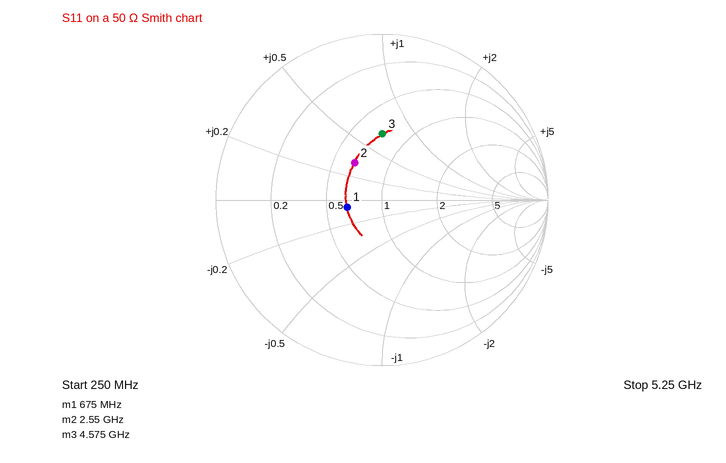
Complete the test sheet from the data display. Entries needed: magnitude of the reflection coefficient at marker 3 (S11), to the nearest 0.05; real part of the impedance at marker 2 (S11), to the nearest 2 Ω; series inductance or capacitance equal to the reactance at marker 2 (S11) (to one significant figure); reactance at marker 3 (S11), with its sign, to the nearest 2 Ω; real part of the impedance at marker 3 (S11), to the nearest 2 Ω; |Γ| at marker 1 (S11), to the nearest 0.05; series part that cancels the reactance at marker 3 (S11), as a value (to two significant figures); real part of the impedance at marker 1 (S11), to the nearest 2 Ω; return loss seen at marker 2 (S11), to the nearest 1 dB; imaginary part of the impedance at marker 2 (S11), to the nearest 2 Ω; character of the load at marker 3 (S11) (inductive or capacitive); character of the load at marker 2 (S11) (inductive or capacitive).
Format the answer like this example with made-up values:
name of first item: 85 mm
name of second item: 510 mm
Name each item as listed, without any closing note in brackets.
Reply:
magnitude of the reflection coefficient at marker 3 (S11), to the nearest 0.05: 0.40
real part of the impedance at marker 2 (S11), to the nearest 2 Ω: 32 Ω
series inductance or capacitance equal to the reactance at marker 2 (S11): 1.0 nH
reactance at marker 3 (S11), with its sign, to the nearest 2 Ω: +34 Ω
real part of the impedance at marker 3 (S11), to the nearest 2 Ω: 36 Ω
|Γ| at marker 1 (S11), to the nearest 0.05: 0.20
series part that cancels the reactance at marker 3 (S11), as a value: 1.0 pF
real part of the impedance at marker 1 (S11), to the nearest 2 Ω: 32 Ω
return loss seen at marker 2 (S11), to the nearest 1 dB: 11 dB
imaginary part of the impedance at marker 2 (S11), to the nearest 2 Ω: +16 Ω
character of the load at marker 3 (S11): inductive
character of the load at marker 2 (S11): inductive
